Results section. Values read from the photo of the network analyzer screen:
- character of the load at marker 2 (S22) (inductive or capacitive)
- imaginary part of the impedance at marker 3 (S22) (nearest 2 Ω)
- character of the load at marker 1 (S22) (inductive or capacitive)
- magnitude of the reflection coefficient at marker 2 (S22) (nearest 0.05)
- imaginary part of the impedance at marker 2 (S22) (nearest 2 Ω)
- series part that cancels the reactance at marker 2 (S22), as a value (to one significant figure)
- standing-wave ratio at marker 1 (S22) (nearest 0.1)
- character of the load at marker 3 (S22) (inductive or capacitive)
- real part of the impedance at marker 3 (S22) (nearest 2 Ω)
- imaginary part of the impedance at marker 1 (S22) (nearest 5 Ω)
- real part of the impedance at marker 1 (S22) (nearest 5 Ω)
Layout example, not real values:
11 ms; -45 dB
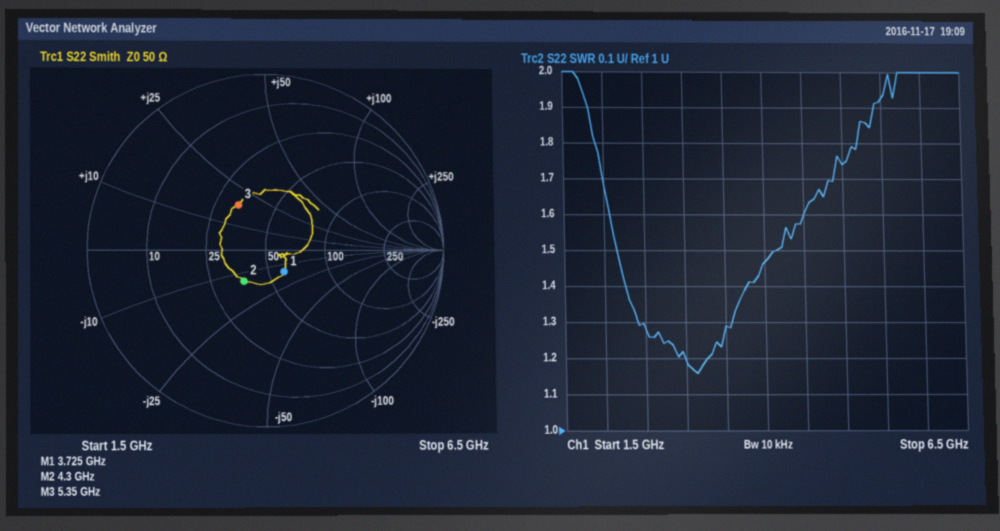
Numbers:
capacitive; +18 Ω; capacitive; 0.20; -14 Ω; 500 pH; 1.4; inductive; 32 Ω; -15 Ω; 60 Ω
